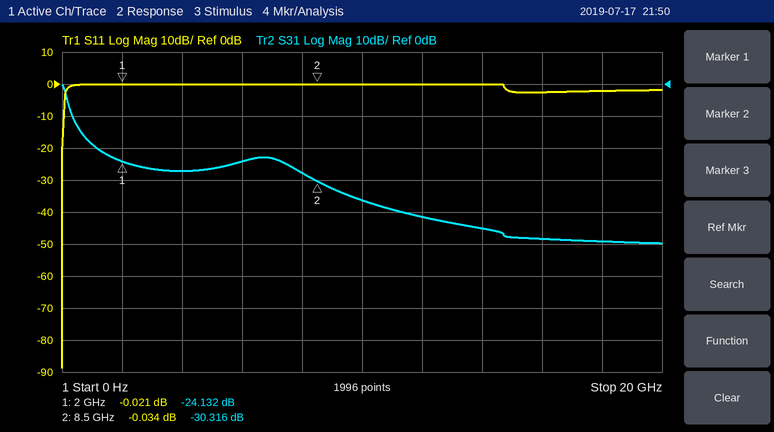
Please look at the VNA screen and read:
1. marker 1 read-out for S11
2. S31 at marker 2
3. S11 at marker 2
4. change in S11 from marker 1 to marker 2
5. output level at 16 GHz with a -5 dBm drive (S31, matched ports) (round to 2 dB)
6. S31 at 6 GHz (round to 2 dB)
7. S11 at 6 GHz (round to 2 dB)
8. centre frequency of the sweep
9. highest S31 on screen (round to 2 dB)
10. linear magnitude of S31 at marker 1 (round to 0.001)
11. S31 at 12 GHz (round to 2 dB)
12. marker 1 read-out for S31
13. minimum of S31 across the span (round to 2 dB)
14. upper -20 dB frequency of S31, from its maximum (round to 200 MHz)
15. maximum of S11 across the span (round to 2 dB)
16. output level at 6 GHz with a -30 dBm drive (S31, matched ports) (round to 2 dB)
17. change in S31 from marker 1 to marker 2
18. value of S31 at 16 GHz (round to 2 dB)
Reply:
-0.021 dB
-30.316 dB
-0.034 dB
-0.013 dB
-54 dBm
-24 dB
0 dB
10 GHz
0 dB
0.062
-42 dB
-24.132 dB
-50 dB
1.2 GHz
0 dB
-54 dBm
-6.184 dB
-48 dB
